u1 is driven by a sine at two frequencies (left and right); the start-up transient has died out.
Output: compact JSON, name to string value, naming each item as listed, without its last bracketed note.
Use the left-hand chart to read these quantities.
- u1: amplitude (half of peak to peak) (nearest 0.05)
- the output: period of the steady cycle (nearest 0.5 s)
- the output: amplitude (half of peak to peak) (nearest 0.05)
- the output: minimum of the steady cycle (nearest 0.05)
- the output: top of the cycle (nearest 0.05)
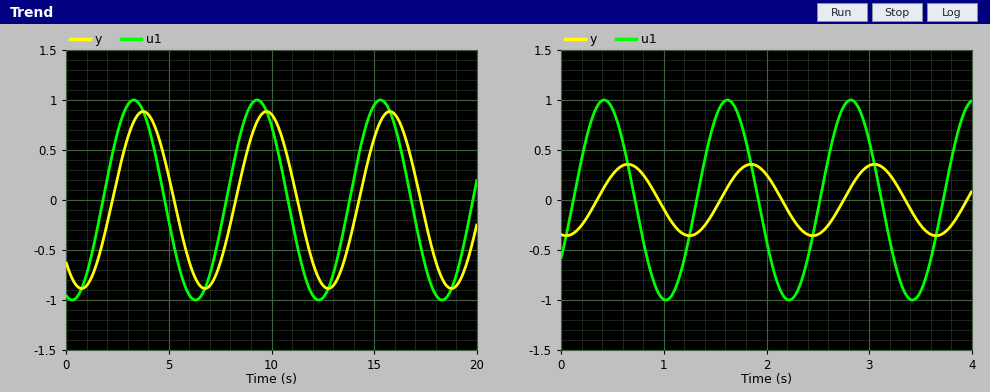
{"u1: amplitude (half of peak to peak)": "1.00", "the output: period of the steady cycle": "6.0 s", "the output: amplitude (half of peak to peak)": "0.90", "the output: minimum of the steady cycle": "-0.90", "the output: top of the cycle": "0.90"}
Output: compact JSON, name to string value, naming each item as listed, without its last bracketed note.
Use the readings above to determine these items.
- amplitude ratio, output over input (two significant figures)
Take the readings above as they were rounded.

{"amplitude ratio, output over input": "0.90"}
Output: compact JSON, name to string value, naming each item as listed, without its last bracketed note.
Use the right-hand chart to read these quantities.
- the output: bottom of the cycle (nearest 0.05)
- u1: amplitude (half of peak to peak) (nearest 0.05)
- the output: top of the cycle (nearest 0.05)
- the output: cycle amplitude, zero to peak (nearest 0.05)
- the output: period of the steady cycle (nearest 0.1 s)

{"the output: bottom of the cycle": "-0.35", "u1: amplitude (half of peak to peak)": "1.00", "the output: top of the cycle": "0.35", "the output: cycle amplitude, zero to peak": "0.35", "the output: period of the steady cycle": "1.2 s"}
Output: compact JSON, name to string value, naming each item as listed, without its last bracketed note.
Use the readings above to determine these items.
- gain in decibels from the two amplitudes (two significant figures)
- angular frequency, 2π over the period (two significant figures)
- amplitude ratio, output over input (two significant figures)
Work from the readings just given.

{"gain in decibels from the two amplitudes": "-9.1 dB", "angular frequency, 2π over the period": "5.2 rad/s", "amplitude ratio, output over input": "0.35"}
